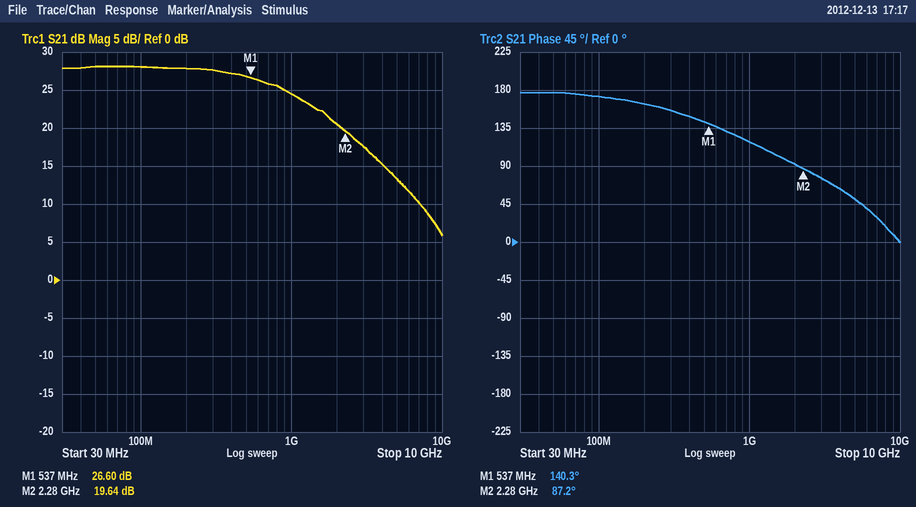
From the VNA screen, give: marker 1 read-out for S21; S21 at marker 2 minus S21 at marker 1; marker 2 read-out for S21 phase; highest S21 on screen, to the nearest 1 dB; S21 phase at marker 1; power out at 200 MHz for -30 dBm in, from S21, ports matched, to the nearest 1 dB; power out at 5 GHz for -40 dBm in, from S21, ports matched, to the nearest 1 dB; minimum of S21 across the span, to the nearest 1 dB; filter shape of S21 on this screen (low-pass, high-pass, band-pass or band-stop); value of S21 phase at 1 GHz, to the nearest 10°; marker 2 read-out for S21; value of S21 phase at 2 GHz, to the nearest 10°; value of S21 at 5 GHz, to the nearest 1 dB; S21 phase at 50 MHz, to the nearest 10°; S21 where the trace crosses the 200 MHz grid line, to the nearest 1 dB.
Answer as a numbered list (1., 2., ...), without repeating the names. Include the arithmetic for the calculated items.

1. 26.60 dB
2. 19.64 − (26.6) = -6.96 dB
3. 87.2°
4. 28 dB
5. 140.3°
6. -30 dBm + (28 dB) = -2 dBm
7. -40 dBm + (13 dB) = -27 dBm
8. 6 dB
9. low-pass
10. 120°
11. 19.64 dB
12. 90°
13. 13 dB
14. 180°
15. 28 dB
